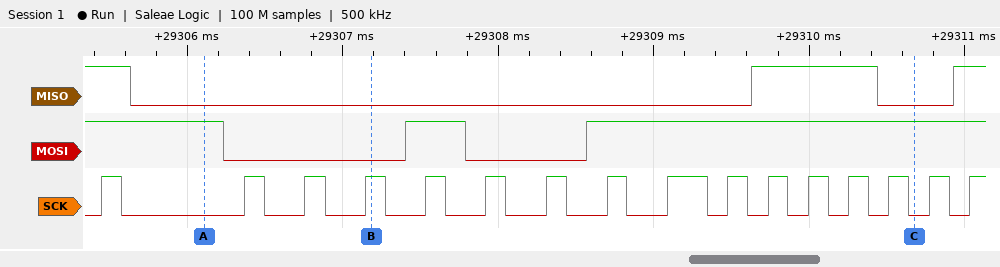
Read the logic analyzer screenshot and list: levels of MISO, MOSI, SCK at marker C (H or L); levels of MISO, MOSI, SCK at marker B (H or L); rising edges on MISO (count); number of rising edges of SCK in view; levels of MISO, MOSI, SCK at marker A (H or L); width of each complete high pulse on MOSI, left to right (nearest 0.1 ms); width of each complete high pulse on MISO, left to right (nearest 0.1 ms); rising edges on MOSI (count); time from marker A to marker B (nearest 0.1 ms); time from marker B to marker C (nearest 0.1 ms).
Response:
MISO=L, MOSI=H, SCK=L
MISO=L, MOSI=L, SCK=H
2
16
MISO=L, MOSI=H, SCK=L
0.4 ms
0.8 ms
2
1.1 ms
3.5 ms
